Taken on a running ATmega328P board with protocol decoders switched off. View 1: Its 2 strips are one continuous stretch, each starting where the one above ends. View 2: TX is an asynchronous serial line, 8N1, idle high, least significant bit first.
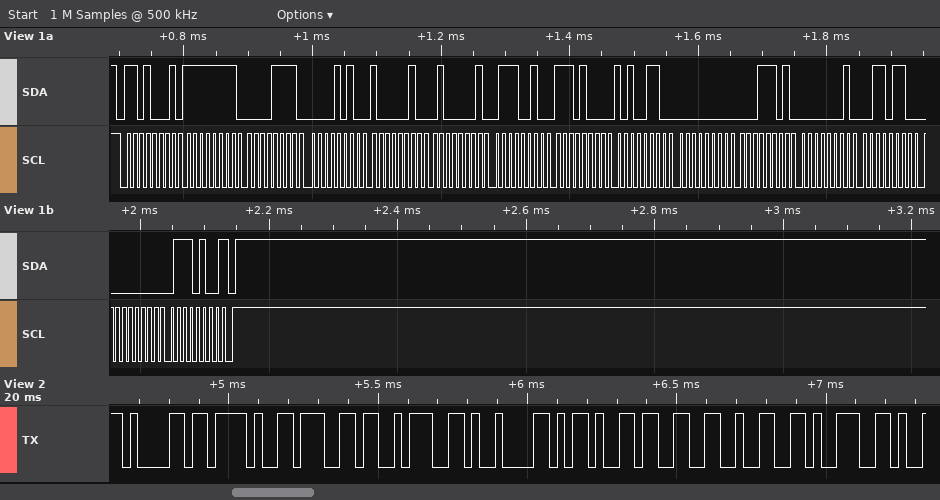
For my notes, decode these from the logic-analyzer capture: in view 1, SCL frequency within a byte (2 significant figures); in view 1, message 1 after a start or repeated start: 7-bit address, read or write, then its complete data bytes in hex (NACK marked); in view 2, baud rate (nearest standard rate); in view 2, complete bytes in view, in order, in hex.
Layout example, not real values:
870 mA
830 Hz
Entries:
100 kHz
0x68 read: FF 0F 0A 82 41 72 E8 A6 00 1D 01 36 00 74 NACK
38400 baud
61 2F 67 3A 09 2D 33 32 39
